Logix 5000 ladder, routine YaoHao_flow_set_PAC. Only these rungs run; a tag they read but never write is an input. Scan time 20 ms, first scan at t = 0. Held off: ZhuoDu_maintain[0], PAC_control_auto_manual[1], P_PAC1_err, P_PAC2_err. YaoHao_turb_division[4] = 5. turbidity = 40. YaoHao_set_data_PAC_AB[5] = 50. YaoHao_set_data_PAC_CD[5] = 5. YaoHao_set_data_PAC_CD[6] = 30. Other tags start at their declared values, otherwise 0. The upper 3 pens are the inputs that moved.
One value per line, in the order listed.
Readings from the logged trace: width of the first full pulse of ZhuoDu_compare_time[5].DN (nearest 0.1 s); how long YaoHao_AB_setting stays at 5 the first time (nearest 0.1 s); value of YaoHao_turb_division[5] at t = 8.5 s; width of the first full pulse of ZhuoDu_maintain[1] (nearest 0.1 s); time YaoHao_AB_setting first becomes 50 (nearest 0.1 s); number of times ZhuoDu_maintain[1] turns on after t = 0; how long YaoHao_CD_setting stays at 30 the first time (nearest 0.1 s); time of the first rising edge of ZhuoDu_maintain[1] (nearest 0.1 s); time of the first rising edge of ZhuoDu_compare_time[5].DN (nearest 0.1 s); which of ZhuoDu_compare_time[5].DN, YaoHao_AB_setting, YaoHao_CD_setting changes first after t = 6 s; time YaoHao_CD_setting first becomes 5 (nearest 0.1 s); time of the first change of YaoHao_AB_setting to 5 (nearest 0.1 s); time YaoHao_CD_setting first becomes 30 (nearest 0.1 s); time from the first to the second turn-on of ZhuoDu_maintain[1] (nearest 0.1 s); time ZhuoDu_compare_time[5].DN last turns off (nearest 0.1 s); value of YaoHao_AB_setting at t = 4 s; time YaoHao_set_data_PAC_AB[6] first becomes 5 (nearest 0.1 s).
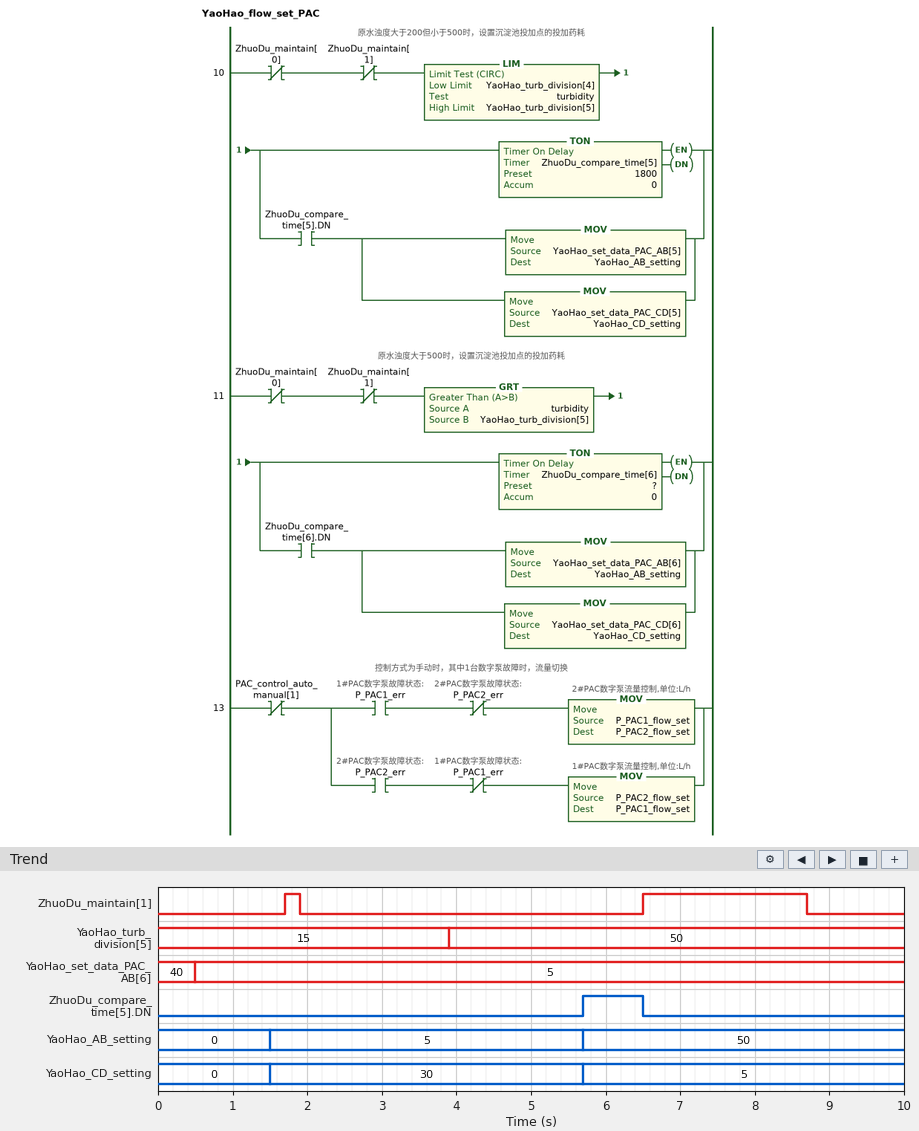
0.8 s
4.2 s
50
0.2 s
5.7 s
2
4.2 s
1.7 s
5.7 s
ZhuoDu_compare_time[5].DN
5.7 s
1.5 s
1.5 s
4.8 s
6.5 s
5
0.5 s
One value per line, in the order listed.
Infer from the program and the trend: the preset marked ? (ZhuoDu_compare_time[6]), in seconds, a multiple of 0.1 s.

1.5 s
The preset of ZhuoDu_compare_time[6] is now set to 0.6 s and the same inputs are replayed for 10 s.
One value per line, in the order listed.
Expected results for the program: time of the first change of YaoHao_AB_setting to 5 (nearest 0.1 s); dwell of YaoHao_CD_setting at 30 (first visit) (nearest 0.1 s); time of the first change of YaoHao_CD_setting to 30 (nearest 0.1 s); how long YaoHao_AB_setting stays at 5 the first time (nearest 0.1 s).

0.6 s
5.1 s
0.6 s
5.1 s
